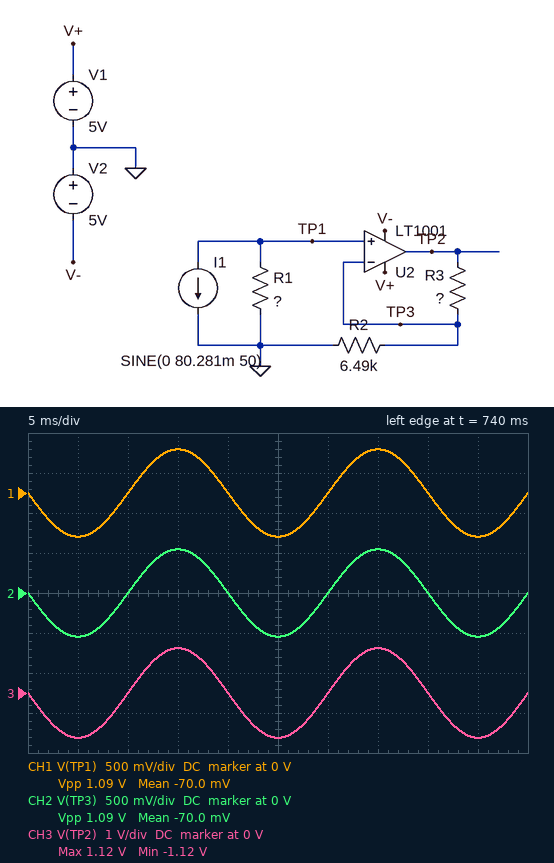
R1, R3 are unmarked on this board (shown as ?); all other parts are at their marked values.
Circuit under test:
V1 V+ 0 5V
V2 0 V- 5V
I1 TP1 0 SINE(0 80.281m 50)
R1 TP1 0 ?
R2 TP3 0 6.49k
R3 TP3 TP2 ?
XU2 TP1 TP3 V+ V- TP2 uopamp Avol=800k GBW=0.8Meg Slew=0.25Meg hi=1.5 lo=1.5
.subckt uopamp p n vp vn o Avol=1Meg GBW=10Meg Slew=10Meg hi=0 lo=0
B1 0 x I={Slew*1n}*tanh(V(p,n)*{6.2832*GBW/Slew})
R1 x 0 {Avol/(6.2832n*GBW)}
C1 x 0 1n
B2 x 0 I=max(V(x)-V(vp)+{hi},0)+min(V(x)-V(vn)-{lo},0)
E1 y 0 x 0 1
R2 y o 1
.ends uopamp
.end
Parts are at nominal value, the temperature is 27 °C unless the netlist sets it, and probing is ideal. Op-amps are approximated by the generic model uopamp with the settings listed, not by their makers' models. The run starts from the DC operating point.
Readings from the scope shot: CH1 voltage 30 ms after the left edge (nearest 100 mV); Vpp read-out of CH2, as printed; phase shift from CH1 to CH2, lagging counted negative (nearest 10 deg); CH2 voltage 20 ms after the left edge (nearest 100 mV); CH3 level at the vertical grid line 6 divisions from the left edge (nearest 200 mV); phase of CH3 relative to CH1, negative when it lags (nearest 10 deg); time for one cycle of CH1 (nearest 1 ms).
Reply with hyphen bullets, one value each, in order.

- 0 V
- 1.09 V
- 0 deg
- 0 V
- 0 V
- 0 deg
- 20 ms
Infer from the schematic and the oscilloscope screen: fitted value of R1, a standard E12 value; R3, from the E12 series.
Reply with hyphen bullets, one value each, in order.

- 6.8 Ω
- 6.8 kΩ
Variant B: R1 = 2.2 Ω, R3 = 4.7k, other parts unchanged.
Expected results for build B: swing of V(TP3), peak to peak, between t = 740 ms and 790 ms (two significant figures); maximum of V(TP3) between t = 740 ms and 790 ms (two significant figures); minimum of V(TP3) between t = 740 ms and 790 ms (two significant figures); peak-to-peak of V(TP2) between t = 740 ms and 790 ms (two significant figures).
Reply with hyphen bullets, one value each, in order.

- 350 mV
- 180 mV
- -180 mV
- 610 mV
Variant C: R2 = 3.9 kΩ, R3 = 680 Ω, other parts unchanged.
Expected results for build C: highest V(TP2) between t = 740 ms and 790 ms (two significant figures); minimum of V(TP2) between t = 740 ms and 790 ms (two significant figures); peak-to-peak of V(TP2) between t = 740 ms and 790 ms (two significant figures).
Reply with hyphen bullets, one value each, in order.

- 640 mV
- -640 mV
- 1.3 V
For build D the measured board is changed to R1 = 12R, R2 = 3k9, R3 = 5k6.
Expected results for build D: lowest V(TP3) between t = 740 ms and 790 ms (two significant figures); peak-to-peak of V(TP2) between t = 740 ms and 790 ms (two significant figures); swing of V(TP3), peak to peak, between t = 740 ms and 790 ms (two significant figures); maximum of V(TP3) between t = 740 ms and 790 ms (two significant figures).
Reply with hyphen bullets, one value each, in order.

- -960 mV
- 4.7 V
- 1.9 V
- 960 mV
